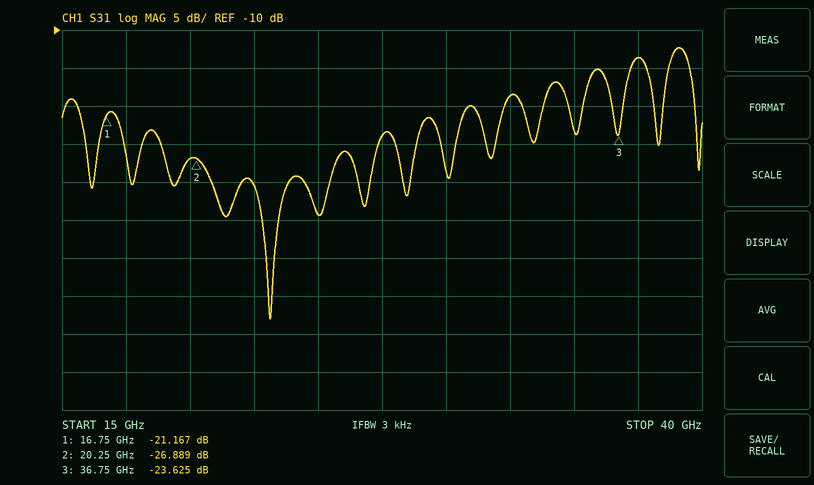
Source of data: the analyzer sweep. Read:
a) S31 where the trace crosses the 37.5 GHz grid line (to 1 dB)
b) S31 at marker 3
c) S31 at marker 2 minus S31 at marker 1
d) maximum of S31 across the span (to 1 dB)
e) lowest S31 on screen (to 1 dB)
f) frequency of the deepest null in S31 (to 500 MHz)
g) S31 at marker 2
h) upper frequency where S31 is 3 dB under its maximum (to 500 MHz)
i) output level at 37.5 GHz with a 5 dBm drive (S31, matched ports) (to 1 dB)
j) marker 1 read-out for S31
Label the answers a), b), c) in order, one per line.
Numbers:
a) -14 dB
b) -23.625 dB
c) -5.722 dB
d) -12 dB
e) -48 dB
f) 23.0 GHz
g) -26.889 dB
h) 39.5 GHz
i) -9 dBm
j) -21.167 dB
